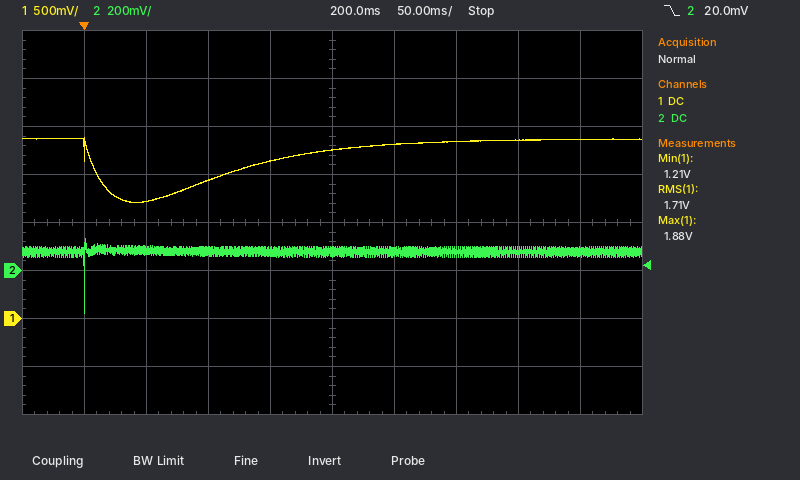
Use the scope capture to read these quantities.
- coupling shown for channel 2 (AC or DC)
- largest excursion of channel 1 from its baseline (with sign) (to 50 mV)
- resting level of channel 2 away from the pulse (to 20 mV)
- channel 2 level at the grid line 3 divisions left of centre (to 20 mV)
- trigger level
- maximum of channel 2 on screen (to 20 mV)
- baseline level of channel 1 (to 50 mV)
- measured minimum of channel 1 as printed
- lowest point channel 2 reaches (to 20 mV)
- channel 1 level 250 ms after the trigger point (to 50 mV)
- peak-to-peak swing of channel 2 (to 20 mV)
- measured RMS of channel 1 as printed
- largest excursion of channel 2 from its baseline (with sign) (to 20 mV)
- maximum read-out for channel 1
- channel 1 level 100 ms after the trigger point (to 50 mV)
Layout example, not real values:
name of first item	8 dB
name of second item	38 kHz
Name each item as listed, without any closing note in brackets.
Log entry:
coupling shown for channel 2	DC
largest excursion of channel 1 from its baseline (with sign)	-650 mV
resting level of channel 2 away from the pulse	80 mV
channel 2 level at the grid line 3 divisions left of centre	80 mV
trigger level	20.0 mV
maximum of channel 2 on screen	140 mV
baseline level of channel 1	1.85 V
measured minimum of channel 1 as printed	1.21 V
lowest point channel 2 reaches	-180 mV
channel 1 level 250 ms after the trigger point	1.80 V
peak-to-peak swing of channel 2	320 mV
measured RMS of channel 1 as printed	1.71 V
largest excursion of channel 2 from its baseline (with sign)	-260 mV
maximum read-out for channel 1	1.88 V
channel 1 level 100 ms after the trigger point	1.45 V
